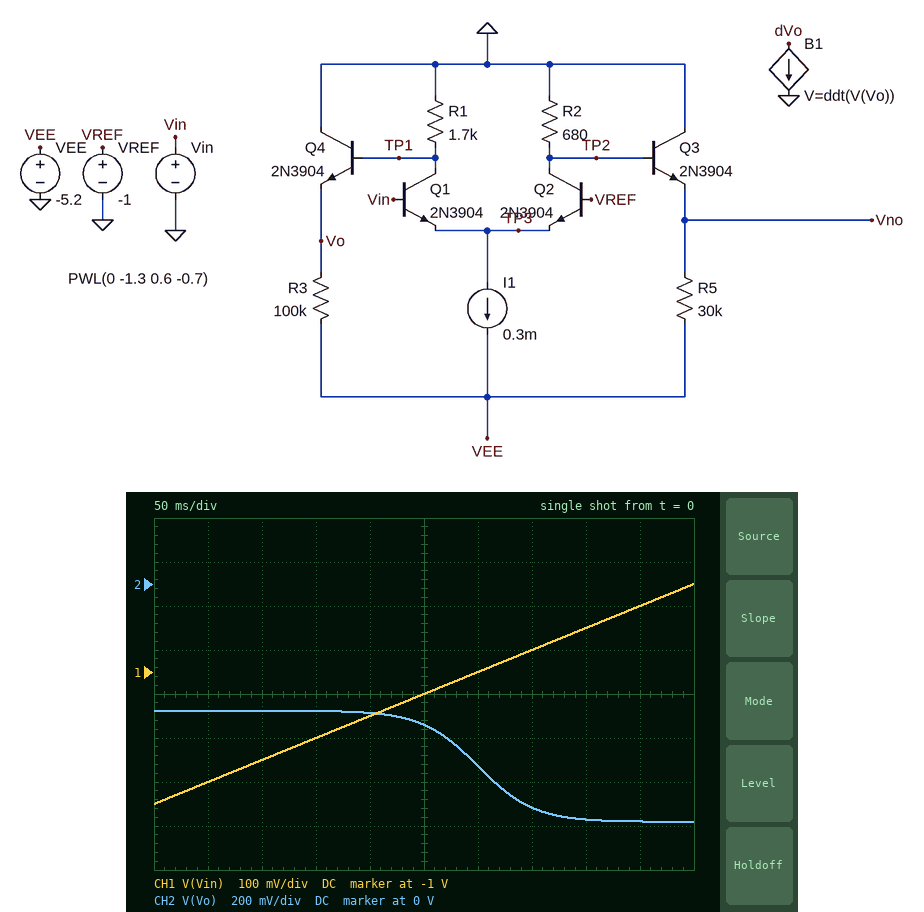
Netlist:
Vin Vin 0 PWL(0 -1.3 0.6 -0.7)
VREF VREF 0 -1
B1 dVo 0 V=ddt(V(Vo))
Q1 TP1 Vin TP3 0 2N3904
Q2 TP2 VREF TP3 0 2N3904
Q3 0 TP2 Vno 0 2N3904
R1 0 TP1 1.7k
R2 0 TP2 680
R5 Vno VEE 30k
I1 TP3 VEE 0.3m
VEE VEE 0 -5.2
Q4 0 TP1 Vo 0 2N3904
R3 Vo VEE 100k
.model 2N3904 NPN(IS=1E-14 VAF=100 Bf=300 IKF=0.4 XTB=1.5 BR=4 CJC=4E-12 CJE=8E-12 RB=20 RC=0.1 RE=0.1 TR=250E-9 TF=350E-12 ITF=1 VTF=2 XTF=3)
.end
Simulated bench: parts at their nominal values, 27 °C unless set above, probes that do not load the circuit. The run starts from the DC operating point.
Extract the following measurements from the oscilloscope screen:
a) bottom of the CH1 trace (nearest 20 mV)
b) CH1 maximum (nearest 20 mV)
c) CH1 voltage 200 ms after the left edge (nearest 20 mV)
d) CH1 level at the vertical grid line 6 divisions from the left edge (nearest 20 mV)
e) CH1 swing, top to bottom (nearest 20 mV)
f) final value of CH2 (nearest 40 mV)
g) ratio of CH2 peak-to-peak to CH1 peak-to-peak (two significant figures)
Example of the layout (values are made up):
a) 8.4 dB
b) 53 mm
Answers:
a) -1.30 V
b) -800 mV
c) -1.10 V
d) -1.00 V
e) 500 mV
f) -1.08 V
g) 1.0
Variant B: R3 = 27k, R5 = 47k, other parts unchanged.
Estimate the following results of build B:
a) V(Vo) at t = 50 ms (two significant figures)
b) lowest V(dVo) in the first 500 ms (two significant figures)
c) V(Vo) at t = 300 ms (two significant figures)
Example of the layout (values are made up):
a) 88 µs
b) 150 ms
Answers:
a) -610 mV
b) -4.9 V
c) -860 mV
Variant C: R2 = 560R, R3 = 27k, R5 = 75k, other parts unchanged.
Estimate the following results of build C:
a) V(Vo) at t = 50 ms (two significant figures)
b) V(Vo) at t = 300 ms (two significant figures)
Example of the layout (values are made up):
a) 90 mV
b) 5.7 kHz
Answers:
a) -610 mV
b) -860 mV
